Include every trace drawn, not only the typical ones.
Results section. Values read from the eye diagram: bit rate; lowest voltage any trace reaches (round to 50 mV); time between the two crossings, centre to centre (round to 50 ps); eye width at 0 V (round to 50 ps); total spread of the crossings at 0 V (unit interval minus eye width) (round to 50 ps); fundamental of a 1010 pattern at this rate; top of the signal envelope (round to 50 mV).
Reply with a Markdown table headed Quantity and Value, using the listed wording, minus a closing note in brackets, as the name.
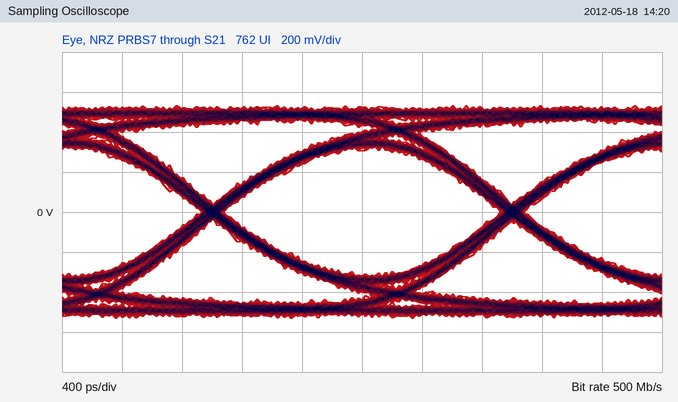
| Quantity | Value |
|---|---|
| bit rate | 500 Mb/s |
| lowest voltage any trace reaches | -550 mV |
| time between the two crossings, centre to centre | 2.00 ns |
| eye width at 0 V | 1.85 ns |
| total spread of the crossings at 0 V (unit interval minus eye width) | 150 ps |
| fundamental of a 1010 pattern at this rate | 250 MHz |
| top of the signal envelope | 550 mV |
